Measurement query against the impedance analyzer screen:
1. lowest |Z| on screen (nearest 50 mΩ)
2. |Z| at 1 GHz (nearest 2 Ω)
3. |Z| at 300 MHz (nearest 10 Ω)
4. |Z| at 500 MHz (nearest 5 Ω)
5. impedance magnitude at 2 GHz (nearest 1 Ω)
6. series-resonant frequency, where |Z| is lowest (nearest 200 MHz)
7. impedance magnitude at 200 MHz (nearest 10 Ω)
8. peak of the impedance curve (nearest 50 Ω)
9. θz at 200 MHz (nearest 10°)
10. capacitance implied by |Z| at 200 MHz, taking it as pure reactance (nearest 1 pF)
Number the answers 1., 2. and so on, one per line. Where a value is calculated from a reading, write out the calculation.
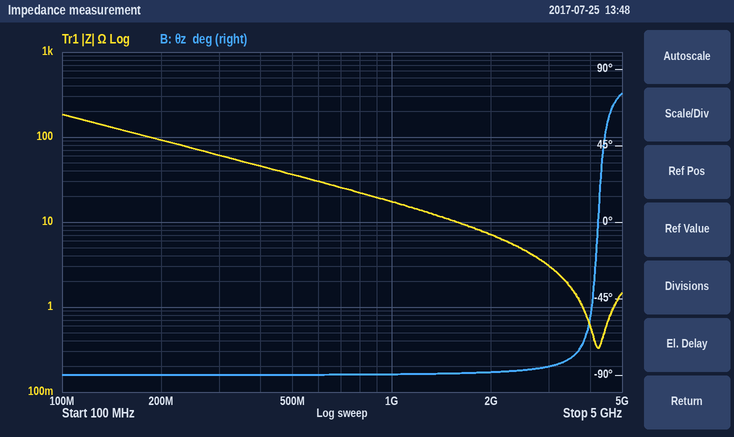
1. 350 mΩ
2. 18 Ω
3. 60 Ω
4. 35 Ω
5. 7 Ω
6. 4.2 GHz
7. 90 Ω
8. 200 Ω
9. -90°
10. C = 1/(2π × 200 MHz × 90 Ω) ≈ 9 pF
